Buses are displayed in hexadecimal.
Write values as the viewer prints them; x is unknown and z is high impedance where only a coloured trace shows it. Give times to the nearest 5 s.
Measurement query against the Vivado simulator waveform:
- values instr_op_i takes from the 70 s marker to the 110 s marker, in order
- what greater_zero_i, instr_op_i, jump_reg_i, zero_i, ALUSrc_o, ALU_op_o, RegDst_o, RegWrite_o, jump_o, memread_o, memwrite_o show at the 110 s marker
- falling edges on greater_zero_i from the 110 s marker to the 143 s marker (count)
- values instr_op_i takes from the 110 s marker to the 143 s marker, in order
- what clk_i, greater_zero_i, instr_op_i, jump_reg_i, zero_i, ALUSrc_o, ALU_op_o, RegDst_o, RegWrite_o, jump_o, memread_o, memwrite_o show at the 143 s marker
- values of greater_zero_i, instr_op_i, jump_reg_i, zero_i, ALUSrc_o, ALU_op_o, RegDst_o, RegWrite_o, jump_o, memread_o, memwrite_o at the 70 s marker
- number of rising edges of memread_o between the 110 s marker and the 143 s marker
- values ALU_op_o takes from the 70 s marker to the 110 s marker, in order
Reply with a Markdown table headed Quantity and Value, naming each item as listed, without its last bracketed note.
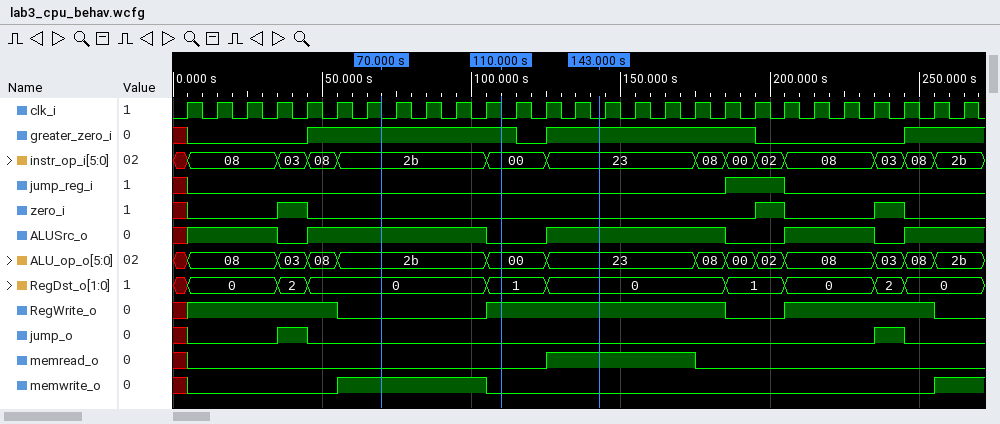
| Quantity | Value |
|---|---|
| values instr_op_i takes from the 70 s marker to the 110 s marker, in order | 2b, 00 |
| what greater_zero_i, instr_op_i, jump_reg_i, zero_i, ALUSrc_o, ALU_op_o, RegDst_o, RegWrite_o, jump_o, memread_o, memwrite_o show at the 110 s marker | greater_zero_i=1, instr_op_i=00, jump_reg_i=0, zero_i=0, ALUSrc_o=0, ALU_op_o=00, RegDst_o=1, RegWrite_o=1, jump_o=0, memread_o=0, memwrite_o=0 |
| falling edges on greater_zero_i from the 110 s marker to the 143 s marker | 1 |
| values instr_op_i takes from the 110 s marker to the 143 s marker, in order | 00, 23 |
| what clk_i, greater_zero_i, instr_op_i, jump_reg_i, zero_i, ALUSrc_o, ALU_op_o, RegDst_o, RegWrite_o, jump_o, memread_o, memwrite_o show at the 143 s marker | clk_i=0, greater_zero_i=1, instr_op_i=23, jump_reg_i=0, zero_i=0, ALUSrc_o=1, ALU_op_o=23, RegDst_o=0, RegWrite_o=1, jump_o=0, memread_o=1, memwrite_o=0 |
| values of greater_zero_i, instr_op_i, jump_reg_i, zero_i, ALUSrc_o, ALU_op_o, RegDst_o, RegWrite_o, jump_o, memread_o, memwrite_o at the 70 s marker | greater_zero_i=1, instr_op_i=2b, jump_reg_i=0, zero_i=0, ALUSrc_o=1, ALU_op_o=2b, RegDst_o=0, RegWrite_o=0, jump_o=0, memread_o=0, memwrite_o=1 |
| number of rising edges of memread_o between the 110 s marker and the 143 s marker | 1 |
| values ALU_op_o takes from the 70 s marker to the 110 s marker, in order | 2b, 00 |
